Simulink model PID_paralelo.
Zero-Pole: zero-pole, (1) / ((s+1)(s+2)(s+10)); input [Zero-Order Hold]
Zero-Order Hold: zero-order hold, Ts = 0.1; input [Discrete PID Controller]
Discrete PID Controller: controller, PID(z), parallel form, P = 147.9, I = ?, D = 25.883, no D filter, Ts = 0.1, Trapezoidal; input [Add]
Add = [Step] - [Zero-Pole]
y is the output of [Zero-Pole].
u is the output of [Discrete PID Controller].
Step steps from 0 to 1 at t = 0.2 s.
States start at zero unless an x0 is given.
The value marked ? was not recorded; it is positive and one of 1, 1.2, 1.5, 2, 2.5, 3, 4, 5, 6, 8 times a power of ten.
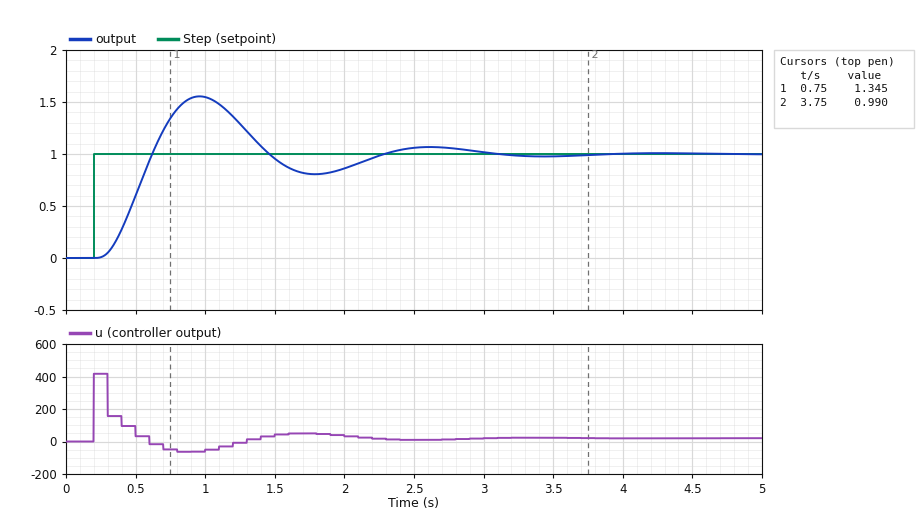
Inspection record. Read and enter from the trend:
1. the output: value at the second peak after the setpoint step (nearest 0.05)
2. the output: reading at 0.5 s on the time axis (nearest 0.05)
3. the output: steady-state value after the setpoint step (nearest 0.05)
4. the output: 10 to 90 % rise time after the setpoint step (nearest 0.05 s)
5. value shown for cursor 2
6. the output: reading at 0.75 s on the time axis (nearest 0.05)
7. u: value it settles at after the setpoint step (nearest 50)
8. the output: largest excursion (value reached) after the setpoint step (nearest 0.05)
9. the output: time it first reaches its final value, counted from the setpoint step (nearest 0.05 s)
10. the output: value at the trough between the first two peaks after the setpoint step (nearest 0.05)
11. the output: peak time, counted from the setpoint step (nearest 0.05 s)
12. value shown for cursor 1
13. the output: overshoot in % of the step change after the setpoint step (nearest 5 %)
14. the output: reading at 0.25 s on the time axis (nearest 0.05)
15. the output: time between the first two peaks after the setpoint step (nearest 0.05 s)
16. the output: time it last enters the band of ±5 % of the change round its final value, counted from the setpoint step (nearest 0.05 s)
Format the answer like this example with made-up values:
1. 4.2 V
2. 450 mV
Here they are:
1. 1.05
2. 0.60
3. 1.00
4. 0.25 s
5. 0.990
6. 1.35
7. 0
8. 1.55
9. 0.40 s
10. 0.80
11. 0.75 s
12. 1.345
13. 55 %
14. 0.00
15. 1.65 s
16. 2.60 s
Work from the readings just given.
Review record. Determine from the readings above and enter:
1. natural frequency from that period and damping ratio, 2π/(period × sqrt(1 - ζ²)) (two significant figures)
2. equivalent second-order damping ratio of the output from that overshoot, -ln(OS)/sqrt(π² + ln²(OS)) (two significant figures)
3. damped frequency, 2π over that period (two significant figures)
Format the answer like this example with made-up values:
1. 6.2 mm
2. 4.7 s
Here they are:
1. 3.9 rad/s
2. 0.19
3. 3.8 rad/s
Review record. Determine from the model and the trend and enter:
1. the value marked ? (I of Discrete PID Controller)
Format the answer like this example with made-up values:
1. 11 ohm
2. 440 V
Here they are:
1. 200
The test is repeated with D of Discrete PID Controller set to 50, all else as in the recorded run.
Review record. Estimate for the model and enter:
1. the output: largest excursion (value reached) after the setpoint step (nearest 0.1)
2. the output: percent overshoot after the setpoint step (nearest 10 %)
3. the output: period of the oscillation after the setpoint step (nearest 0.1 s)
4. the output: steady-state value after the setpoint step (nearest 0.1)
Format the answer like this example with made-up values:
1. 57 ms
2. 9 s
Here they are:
1. 1.4
2. 40 %
3. 1.0 s
4. 1.0
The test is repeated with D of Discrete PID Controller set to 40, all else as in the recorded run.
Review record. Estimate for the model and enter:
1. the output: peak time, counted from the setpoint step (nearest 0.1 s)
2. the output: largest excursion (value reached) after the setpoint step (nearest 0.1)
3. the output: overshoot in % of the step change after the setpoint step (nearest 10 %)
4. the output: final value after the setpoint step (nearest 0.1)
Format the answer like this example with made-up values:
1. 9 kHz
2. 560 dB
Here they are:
1. 0.6 s
2. 1.4
3. 40 %
4. 1.0
